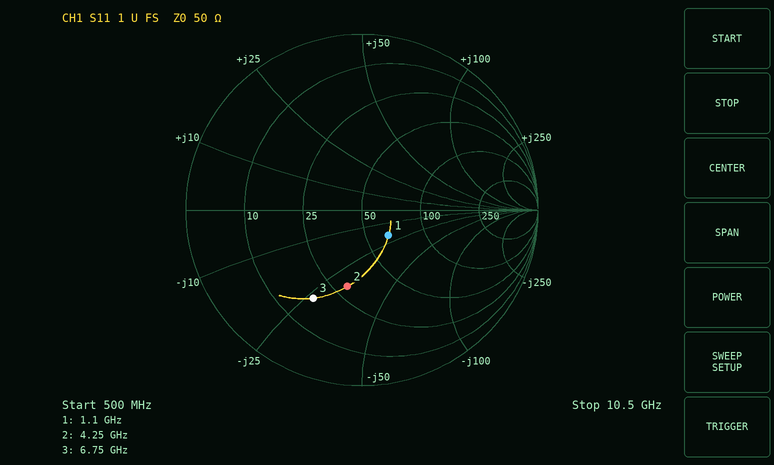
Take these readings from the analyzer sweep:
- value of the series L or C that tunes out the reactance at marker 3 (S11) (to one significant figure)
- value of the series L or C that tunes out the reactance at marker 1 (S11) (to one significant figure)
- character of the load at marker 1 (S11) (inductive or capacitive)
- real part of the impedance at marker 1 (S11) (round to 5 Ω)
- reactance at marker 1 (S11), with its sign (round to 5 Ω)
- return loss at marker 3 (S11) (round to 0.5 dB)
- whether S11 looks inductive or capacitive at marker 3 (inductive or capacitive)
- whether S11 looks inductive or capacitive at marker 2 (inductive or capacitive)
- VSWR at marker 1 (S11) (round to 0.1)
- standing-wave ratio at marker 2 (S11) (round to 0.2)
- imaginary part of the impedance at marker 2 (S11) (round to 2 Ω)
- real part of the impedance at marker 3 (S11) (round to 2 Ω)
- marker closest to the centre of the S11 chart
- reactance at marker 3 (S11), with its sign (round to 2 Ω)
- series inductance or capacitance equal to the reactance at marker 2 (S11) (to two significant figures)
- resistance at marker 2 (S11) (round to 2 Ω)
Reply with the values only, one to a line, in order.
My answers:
600 pH
3 nH
capacitive
65 Ω
-20 Ω
5.0 dB
capacitive
capacitive
1.5
2.6
-32 Ω
18 Ω
marker 1
-26 Ω
1.2 pF
30 Ω
